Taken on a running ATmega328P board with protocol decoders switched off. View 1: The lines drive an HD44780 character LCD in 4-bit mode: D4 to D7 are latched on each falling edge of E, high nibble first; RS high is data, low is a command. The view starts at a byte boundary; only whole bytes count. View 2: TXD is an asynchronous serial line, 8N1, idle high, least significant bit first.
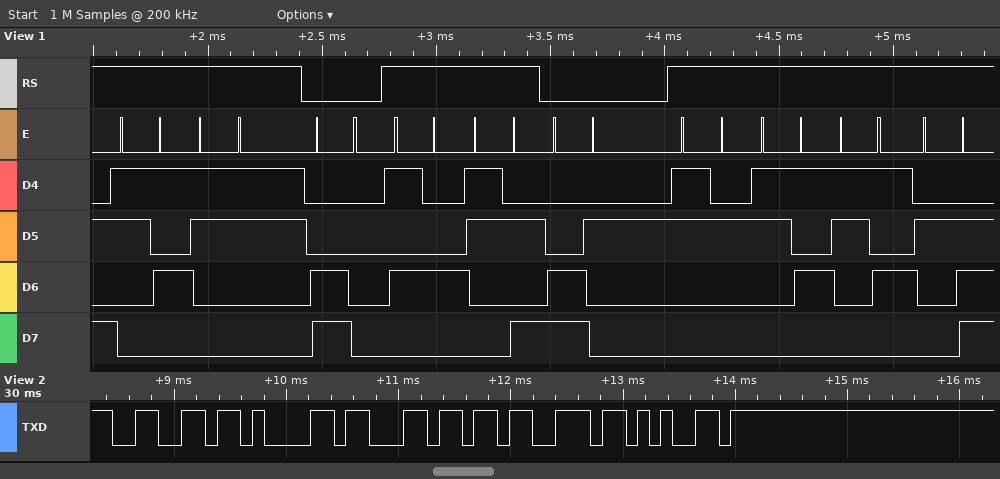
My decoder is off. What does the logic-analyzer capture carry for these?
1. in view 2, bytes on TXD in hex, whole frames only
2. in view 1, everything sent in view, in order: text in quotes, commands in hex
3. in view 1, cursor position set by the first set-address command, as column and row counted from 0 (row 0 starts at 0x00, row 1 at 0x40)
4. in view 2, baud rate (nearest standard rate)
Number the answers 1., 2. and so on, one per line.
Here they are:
1. 66 61 6C 73 65
2. "53" 0xC0 "T:" 0xC2 "255."
3. column 0, row 1
4. 9600 baud
